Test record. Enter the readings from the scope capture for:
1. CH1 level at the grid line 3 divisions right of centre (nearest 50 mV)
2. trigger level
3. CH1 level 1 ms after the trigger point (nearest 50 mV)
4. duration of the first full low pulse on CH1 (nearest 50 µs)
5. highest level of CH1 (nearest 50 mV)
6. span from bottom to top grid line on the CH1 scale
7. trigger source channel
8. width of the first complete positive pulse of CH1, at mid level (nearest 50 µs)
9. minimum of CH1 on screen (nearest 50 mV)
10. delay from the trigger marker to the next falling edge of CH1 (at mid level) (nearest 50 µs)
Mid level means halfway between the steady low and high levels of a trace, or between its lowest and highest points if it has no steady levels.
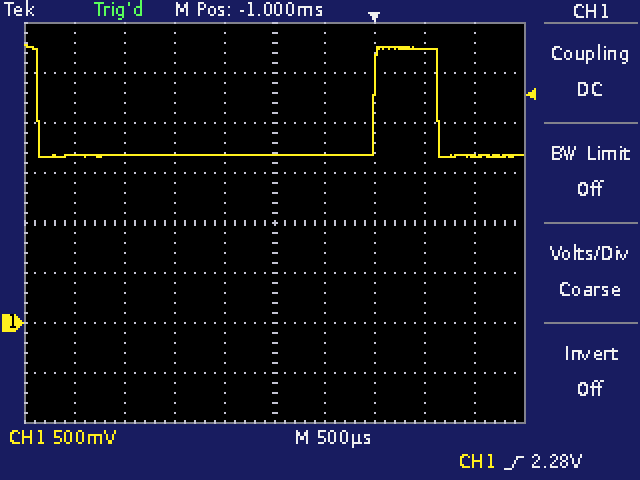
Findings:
2.75 V
2.28 V
1.65 V
3.35 ms
2.80 V
4 V
CH1
650 µs
1.65 V
650 µs
